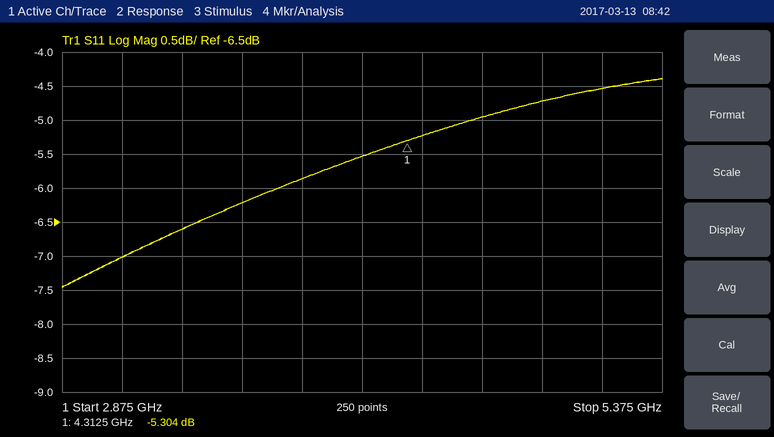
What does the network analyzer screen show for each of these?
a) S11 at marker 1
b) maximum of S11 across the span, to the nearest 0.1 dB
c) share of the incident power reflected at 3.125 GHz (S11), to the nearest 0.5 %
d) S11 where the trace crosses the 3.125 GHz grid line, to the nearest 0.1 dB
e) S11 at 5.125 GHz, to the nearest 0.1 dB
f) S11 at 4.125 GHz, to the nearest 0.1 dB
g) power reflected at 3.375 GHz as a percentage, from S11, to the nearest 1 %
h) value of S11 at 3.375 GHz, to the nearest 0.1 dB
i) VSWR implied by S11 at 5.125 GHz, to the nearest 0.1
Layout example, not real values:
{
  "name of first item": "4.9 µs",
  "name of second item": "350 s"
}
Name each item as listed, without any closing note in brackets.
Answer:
{
  "S11 at marker 1": "-5.304 dB",
  "maximum of S11 across the span, to the nearest 0.1 dB": "-4.4 dB",
  "share of the incident power reflected at 3.125 GHz (S11), to the nearest 0.5 %": "20.0 %",
  "S11 where the trace crosses the 3.125 GHz grid line, to the nearest 0.1 dB": "-7.0 dB",
  "S11 at 5.125 GHz, to the nearest 0.1 dB": "-4.5 dB",
  "S11 at 4.125 GHz, to the nearest 0.1 dB": "-5.5 dB",
  "power reflected at 3.375 GHz as a percentage, from S11, to the nearest 1 %": "22 %",
  "value of S11 at 3.375 GHz, to the nearest 0.1 dB": "-6.6 dB",
  "VSWR implied by S11 at 5.125 GHz, to the nearest 0.1": "3.9"
}
